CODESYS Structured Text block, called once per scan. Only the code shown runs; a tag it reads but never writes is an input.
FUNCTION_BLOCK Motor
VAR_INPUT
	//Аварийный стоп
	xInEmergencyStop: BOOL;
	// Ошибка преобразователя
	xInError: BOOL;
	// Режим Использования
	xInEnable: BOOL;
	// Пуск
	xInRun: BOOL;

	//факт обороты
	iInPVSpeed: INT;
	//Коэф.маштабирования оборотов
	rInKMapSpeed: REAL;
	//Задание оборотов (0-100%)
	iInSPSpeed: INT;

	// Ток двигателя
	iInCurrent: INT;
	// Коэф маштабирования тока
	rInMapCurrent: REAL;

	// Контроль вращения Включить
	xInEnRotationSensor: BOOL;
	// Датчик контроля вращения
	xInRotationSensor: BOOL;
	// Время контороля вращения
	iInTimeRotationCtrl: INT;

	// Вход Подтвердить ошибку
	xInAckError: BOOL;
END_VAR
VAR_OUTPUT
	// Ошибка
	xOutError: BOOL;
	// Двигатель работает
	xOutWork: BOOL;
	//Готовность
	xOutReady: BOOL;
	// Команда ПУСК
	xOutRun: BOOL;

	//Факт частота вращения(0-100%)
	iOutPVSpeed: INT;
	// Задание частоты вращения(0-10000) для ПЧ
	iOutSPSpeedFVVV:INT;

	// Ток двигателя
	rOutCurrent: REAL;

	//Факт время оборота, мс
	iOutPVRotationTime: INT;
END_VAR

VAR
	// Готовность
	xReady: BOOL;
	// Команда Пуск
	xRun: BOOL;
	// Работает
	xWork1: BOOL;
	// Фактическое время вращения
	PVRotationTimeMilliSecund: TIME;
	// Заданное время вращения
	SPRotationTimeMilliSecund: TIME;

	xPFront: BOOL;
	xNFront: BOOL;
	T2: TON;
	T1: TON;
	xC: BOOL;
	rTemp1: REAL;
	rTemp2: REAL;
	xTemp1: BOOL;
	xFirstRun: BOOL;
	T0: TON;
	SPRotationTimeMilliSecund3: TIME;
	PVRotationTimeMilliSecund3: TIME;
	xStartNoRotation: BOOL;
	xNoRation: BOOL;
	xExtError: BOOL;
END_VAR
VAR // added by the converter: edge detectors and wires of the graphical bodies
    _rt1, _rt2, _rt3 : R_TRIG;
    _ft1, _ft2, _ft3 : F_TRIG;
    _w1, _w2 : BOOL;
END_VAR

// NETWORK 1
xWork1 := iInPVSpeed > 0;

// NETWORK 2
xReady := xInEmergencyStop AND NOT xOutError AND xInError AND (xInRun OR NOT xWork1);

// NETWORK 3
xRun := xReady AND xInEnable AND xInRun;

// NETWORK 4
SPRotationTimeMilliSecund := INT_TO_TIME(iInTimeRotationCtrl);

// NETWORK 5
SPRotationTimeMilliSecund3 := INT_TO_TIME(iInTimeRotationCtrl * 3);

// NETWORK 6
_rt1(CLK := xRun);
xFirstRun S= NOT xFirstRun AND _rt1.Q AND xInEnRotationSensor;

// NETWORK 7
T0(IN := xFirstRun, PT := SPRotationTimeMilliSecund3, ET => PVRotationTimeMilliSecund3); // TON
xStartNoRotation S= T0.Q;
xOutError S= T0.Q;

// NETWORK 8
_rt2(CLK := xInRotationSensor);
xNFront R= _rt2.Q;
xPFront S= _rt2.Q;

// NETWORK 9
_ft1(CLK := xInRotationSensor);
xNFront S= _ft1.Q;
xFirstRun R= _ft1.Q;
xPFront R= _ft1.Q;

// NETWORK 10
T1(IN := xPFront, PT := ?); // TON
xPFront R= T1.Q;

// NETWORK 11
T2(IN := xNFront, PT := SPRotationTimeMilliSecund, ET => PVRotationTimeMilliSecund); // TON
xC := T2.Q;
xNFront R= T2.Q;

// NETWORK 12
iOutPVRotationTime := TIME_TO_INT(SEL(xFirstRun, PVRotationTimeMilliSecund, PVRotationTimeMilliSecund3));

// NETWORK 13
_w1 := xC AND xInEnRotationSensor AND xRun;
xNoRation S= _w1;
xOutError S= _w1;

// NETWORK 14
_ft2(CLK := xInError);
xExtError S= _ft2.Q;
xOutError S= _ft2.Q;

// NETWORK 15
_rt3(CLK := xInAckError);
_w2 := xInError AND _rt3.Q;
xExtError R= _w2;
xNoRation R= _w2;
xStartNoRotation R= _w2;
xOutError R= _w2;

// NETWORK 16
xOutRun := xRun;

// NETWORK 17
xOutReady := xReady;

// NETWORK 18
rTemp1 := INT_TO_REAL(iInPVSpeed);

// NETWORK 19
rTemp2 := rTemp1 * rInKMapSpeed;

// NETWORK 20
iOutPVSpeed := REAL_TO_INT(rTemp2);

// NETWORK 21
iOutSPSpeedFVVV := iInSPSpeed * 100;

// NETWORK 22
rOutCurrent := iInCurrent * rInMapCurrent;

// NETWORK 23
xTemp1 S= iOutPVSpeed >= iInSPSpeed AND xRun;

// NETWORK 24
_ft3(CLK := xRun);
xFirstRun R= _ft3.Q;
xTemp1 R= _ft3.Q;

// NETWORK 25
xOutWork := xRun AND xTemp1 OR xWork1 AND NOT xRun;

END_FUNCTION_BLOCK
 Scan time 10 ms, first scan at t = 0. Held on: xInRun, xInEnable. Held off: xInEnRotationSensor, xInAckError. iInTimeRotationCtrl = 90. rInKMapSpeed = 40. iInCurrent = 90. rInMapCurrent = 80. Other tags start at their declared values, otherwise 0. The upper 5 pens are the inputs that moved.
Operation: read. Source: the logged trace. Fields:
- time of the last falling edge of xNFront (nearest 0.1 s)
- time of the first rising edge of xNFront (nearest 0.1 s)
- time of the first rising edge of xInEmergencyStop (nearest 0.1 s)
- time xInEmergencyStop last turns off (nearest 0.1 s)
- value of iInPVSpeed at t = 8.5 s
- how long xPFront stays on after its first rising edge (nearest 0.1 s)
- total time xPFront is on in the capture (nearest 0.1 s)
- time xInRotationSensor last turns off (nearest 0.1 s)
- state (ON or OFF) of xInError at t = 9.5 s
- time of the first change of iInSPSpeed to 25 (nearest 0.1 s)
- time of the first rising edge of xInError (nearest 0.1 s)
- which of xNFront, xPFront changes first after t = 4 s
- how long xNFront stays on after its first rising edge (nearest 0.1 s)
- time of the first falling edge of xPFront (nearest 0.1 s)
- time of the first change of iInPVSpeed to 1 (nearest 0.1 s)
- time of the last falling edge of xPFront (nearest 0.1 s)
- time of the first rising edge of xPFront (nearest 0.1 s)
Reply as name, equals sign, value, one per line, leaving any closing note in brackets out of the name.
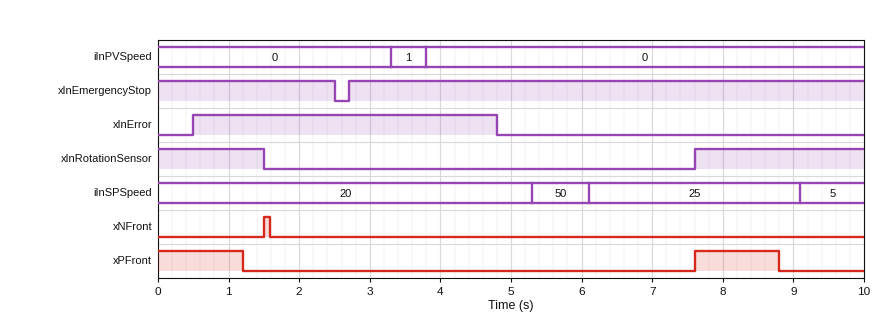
time of the last falling edge of xNFront = 1.6 s
time of the first rising edge of xNFront = 1.5 s
time of the first rising edge of xInEmergencyStop = 2.7 s
time xInEmergencyStop last turns off = 2.5 s
value of iInPVSpeed at t = 8.5 s = 0
how long xPFront stays on after its first rising edge = 1.2 s
total time xPFront is on in the capture = 2.4 s
time xInRotationSensor last turns off = 1.5 s
state (ON or OFF) of xInError at t = 9.5 s = OFF
time of the first change of iInSPSpeed to 25 = 6.1 s
time of the first rising edge of xInError = 0.5 s
which of xNFront, xPFront changes first after t = 4 s = xPFront
how long xNFront stays on after its first rising edge = 0.1 s
time of the first falling edge of xPFront = 1.2 s
time of the first change of iInPVSpeed to 1 = 3.3 s
time of the last falling edge of xPFront = 8.8 s
time of the first rising edge of xPFront = 7.6 s
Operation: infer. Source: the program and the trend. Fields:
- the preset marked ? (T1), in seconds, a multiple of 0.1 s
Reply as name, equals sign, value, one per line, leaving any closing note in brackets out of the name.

the preset marked ? (T1), in seconds, a multiple of 0.1 s = 1.2 s
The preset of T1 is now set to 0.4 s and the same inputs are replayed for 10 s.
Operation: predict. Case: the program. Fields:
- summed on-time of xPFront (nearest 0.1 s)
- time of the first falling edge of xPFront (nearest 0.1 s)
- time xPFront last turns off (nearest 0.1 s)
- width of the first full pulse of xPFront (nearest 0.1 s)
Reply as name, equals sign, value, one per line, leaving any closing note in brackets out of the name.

summed on-time of xPFront = 0.8 s
time of the first falling edge of xPFront = 0.4 s
time xPFront last turns off = 8.0 s
width of the first full pulse of xPFront = 0.4 s
